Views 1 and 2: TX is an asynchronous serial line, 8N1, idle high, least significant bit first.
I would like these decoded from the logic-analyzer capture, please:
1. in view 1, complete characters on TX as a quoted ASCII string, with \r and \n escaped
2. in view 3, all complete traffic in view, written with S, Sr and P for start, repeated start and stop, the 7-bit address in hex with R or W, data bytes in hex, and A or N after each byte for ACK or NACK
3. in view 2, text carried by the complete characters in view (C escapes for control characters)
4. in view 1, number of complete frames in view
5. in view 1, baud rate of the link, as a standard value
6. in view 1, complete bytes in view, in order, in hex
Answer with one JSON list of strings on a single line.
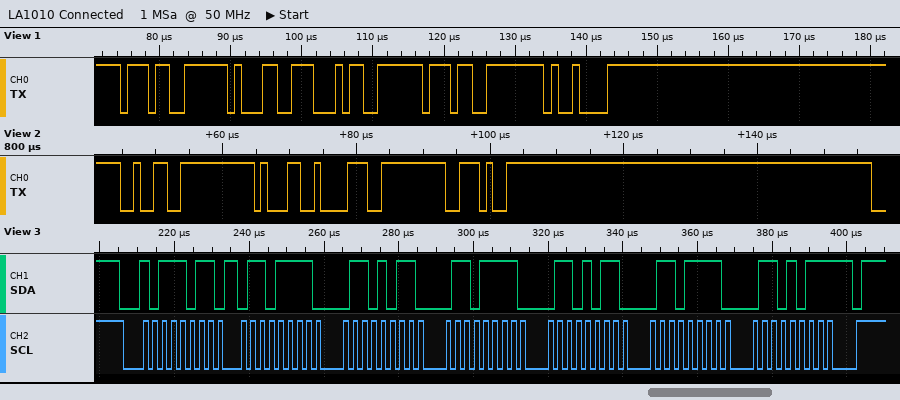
["\"7147\\t\"", "S 5DR A 6F A 6B A 6F A 6B A 6F A 6B N P", "\"218.\"", "5", "1000000 baud", "37 31 34 37 09"]
